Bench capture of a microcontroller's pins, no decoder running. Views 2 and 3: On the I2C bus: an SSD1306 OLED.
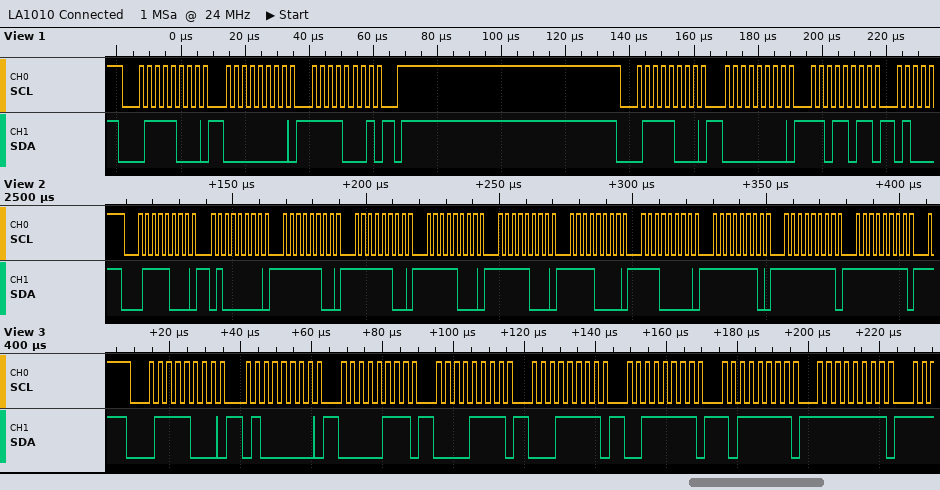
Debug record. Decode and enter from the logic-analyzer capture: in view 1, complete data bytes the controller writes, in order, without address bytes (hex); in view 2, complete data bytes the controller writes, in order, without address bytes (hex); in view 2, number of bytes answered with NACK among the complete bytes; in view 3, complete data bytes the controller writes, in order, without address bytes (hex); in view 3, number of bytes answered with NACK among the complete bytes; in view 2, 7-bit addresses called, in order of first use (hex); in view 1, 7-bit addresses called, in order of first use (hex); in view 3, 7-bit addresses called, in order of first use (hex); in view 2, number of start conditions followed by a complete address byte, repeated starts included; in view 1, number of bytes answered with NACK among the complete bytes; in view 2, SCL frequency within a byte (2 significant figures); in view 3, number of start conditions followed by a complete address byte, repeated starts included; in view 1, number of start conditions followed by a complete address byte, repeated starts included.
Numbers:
00 F1 00 DB
40 FC FC F8 F8 F0 E0 FE FF FF
0
40 07 0F 1F 3F BF FF
0
0x3C
0x3C
0x3C
1
0
400 kHz
1
2
